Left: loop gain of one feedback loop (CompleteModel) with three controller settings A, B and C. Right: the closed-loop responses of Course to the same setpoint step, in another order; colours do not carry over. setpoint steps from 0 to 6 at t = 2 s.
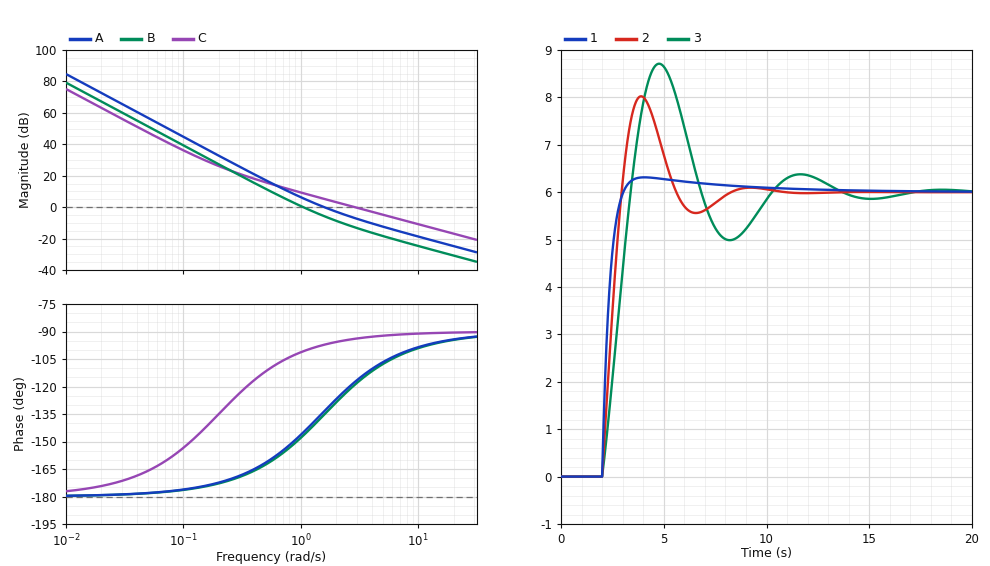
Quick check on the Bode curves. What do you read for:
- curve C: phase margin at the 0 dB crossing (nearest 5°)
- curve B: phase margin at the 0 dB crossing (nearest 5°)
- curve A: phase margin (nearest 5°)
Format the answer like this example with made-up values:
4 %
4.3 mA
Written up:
85°
35°
45°
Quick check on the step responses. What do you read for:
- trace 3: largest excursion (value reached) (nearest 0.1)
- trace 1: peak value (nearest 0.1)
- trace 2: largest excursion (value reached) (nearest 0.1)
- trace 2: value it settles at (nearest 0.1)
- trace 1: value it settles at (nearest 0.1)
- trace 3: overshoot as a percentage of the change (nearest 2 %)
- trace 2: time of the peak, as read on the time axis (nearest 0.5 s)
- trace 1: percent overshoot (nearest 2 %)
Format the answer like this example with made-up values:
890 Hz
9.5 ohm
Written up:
8.7
6.3
8.0
6.0
6.0
46 %
4.0 s
6 %
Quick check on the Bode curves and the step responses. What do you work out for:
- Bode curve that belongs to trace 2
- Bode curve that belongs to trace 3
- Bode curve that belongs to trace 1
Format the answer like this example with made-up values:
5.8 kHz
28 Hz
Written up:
A
B
C
